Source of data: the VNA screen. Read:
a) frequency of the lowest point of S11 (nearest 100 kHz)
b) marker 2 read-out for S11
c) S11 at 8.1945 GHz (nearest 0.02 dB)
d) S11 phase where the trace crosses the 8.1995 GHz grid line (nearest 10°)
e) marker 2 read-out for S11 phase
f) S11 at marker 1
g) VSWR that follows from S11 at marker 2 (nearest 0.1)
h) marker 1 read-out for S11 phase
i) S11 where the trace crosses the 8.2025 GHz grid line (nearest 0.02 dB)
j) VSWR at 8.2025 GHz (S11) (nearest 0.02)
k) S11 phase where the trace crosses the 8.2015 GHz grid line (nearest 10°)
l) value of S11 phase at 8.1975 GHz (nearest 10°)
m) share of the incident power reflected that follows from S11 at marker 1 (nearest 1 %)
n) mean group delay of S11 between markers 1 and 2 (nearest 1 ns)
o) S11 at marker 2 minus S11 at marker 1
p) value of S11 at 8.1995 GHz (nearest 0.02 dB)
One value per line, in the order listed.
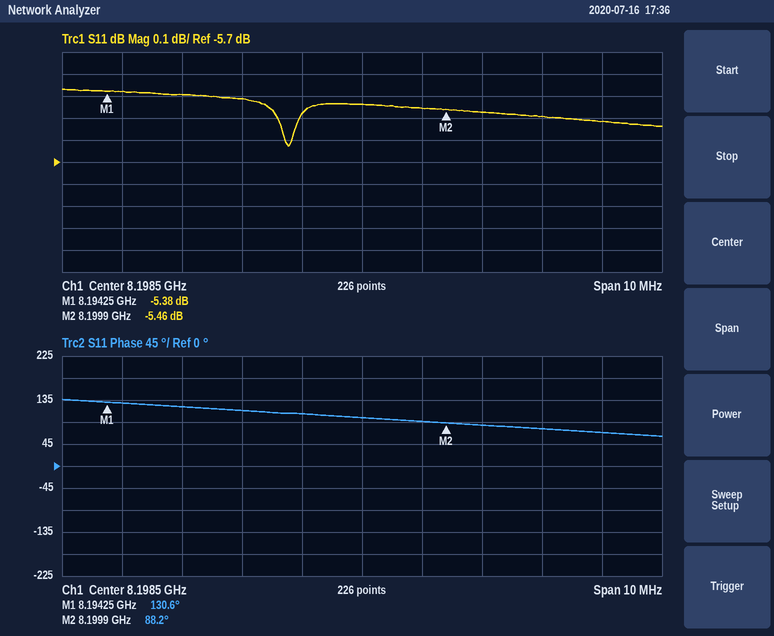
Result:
8.1973 GHz
-5.46 dB
-5.38 dB
90°
88.2°
-5.38 dB
3.3
130.6°
-5.52 dB
3.26
80°
110°
29 %
21 ns
-0.08 dB
-5.46 dB
